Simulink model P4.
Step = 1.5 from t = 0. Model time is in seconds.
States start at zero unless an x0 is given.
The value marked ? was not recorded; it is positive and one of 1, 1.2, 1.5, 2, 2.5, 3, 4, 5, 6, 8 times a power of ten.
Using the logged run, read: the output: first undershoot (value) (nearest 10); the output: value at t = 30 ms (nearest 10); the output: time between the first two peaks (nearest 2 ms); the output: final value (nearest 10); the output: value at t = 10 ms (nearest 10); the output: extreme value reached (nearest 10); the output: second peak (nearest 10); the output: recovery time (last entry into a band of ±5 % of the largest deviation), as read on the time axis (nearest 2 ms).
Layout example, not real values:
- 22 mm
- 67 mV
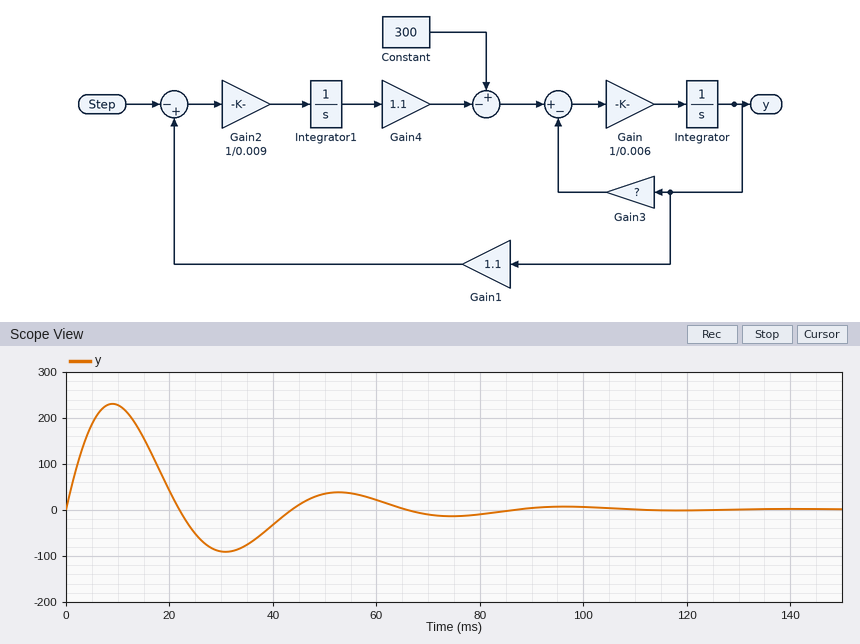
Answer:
- -90
- -90
- 44 ms
- 0
- 230
- 230
- 40
- 80 ms
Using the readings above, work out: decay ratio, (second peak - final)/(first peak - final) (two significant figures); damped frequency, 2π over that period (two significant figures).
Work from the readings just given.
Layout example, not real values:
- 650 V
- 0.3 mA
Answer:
- 0.17
- 0.14 rad/ms
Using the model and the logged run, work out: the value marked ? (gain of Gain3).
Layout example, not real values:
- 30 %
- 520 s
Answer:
- 0.5
